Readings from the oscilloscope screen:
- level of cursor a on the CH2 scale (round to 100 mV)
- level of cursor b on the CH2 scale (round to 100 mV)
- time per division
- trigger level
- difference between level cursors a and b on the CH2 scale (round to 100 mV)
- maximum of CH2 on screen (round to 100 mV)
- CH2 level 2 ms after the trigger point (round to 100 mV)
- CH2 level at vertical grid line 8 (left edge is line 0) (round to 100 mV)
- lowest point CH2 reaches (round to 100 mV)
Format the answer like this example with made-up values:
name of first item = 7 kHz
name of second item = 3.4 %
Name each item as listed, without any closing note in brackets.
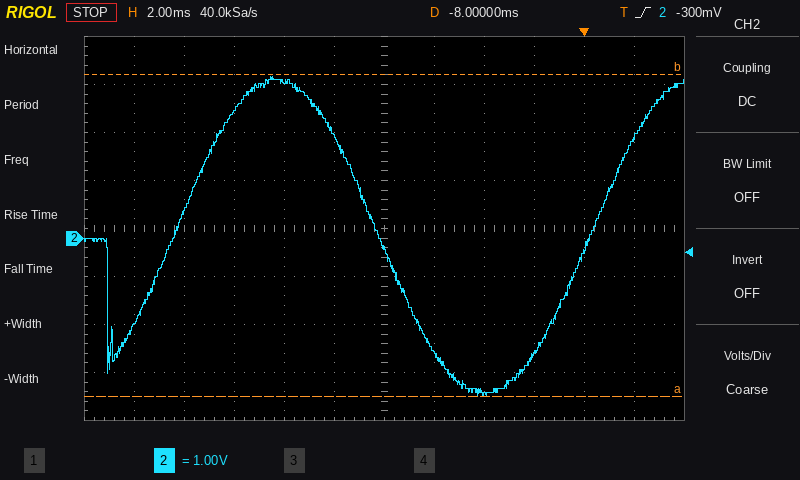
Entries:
level of cursor a on the CH2 scale = -3.3 V
level of cursor b on the CH2 scale = 3.4 V
time per division = 2 ms
trigger level = -300 mV
difference between level cursors a and b on the CH2 scale = 6.7 V
maximum of CH2 on screen = 3.4 V
CH2 level 2 ms after the trigger point = 2.1 V
CH2 level at vertical grid line 8 (left edge is line 0) = -3.2 V
lowest point CH2 reaches = -3.3 V
